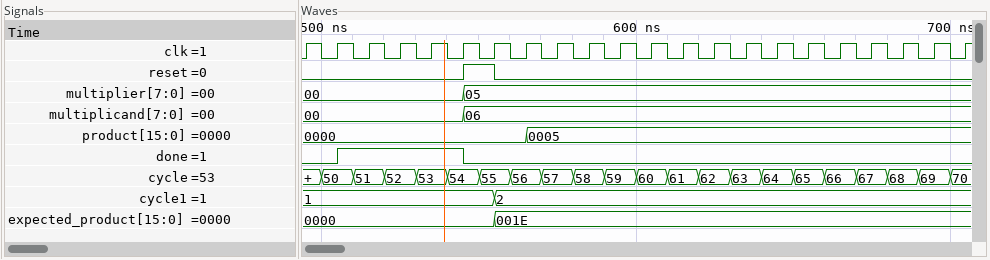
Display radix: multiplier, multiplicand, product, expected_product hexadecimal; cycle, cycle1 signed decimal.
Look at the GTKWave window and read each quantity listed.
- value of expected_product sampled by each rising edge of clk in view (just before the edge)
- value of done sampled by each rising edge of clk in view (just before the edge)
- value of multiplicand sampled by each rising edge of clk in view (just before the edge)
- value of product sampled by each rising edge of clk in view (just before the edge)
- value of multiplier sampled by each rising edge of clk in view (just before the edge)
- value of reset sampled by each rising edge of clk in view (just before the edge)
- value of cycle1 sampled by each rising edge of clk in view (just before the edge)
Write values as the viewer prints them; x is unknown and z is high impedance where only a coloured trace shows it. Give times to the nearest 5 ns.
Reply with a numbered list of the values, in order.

1. 0000, 0000, 0000, 0000, 0000, 0000, 0000, 001E, 001E, 001E, 001E, 001E, 001E, 001E, 001E, 001E, 001E, 001E, 001E, 001E, 001E, 001E
2. 0 0 1 1 1 1 0 0 0 0 0 0 0 0 0 0 0 0 0 0 0 0
3. 00, 00, 00, 00, 00, 00, 06, 06, 06, 06, 06, 06, 06, 06, 06, 06, 06, 06, 06, 06, 06, 06
4. 0000, 0000, 0000, 0000, 0000, 0000, 0000, 0000, 0005, 0005, 0005, 0005, 0005, 0005, 0005, 0005, 0005, 0005, 0005, 0005, 0005, 0005
5. 00, 00, 00, 00, 00, 00, 05, 05, 05, 05, 05, 05, 05, 05, 05, 05, 05, 05, 05, 05, 05, 05
6. 0 0 0 0 0 0 1 0 0 0 0 0 0 0 0 0 0 0 0 0 0 0
7. 1, 1, 1, 1, 1, 1, 1, 2, 2, 2, 2, 2, 2, 2, 2, 2, 2, 2, 2, 2, 2, 2
